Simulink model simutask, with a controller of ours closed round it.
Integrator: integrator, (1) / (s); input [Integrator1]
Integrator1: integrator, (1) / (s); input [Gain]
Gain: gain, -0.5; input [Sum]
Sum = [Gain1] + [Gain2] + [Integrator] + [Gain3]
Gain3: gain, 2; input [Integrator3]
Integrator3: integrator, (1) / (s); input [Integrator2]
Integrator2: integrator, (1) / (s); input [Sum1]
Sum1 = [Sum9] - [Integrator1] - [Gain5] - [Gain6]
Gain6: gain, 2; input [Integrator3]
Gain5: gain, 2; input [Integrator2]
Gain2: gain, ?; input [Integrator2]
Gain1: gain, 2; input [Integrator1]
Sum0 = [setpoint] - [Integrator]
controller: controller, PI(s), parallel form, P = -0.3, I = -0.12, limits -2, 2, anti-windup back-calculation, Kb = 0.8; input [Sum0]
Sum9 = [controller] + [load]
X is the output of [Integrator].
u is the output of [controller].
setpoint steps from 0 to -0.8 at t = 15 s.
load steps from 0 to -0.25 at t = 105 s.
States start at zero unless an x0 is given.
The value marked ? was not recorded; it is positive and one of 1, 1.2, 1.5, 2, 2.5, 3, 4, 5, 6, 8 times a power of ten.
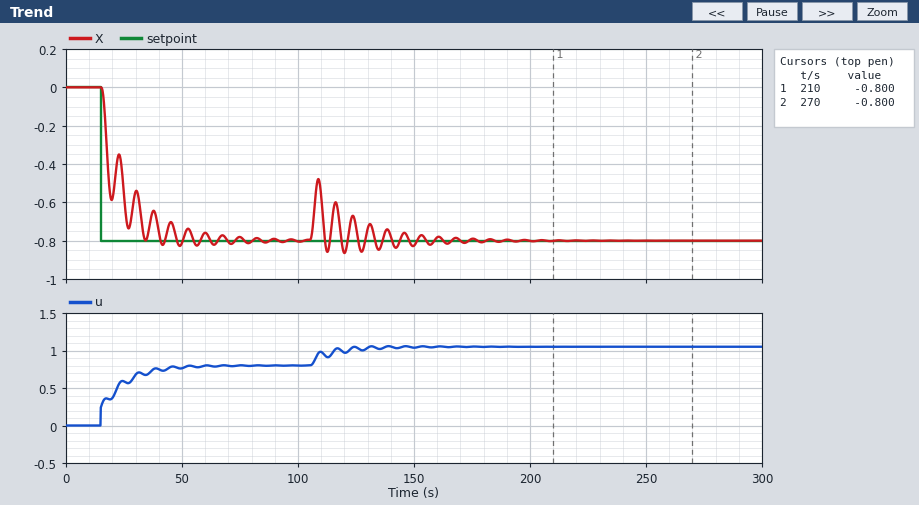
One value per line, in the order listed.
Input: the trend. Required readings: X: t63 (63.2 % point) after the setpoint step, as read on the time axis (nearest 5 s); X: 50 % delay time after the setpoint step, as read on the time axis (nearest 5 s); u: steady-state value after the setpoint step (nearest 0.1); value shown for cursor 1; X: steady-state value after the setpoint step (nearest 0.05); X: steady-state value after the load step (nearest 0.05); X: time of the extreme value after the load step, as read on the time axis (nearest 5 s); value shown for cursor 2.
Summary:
20 s
20 s
0.8
-0.800
-0.80
-0.80
110 s
-0.800
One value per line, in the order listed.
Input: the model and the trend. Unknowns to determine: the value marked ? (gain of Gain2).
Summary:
3
